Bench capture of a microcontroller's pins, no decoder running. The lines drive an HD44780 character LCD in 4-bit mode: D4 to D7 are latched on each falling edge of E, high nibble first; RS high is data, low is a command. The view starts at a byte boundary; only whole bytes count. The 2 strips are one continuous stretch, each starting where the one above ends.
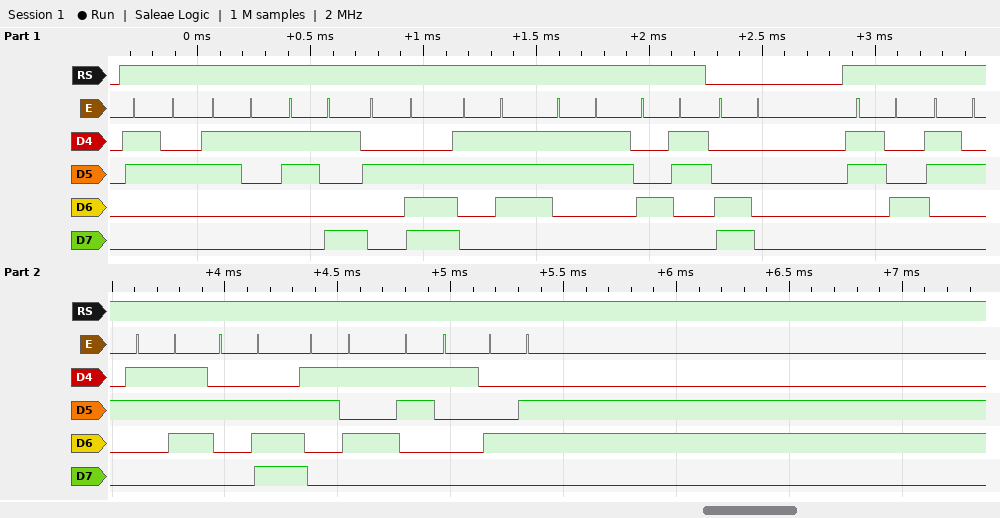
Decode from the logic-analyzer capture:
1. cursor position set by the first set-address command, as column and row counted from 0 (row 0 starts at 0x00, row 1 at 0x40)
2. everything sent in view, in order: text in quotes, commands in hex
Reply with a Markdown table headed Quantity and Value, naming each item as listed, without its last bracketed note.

| Quantity | Value |
|---|---|
| cursor position set by the first set-address command, as column and row counted from 0 | column 0, row 1 |
| everything sent in view, in order: text in quotes, commands in hex | "219.73C" 0xC0 "427.51F" |
